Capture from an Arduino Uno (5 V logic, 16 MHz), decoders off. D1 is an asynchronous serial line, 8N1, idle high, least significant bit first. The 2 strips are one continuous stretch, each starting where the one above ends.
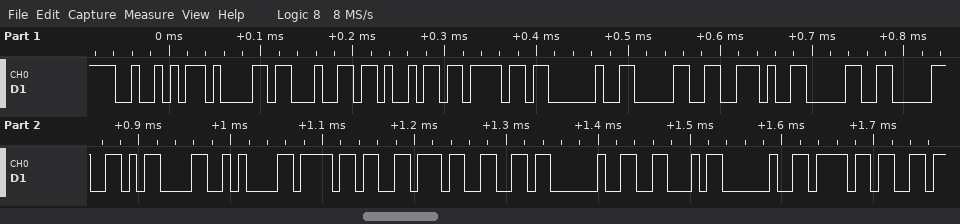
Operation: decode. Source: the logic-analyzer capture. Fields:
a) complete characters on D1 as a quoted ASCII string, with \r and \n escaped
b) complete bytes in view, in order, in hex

"Radio 0.00\r\novf F o"
52 61 64 69 6F 20 30 2E 30 30 0D 0A 6F 76 66 20 46 20 6F
